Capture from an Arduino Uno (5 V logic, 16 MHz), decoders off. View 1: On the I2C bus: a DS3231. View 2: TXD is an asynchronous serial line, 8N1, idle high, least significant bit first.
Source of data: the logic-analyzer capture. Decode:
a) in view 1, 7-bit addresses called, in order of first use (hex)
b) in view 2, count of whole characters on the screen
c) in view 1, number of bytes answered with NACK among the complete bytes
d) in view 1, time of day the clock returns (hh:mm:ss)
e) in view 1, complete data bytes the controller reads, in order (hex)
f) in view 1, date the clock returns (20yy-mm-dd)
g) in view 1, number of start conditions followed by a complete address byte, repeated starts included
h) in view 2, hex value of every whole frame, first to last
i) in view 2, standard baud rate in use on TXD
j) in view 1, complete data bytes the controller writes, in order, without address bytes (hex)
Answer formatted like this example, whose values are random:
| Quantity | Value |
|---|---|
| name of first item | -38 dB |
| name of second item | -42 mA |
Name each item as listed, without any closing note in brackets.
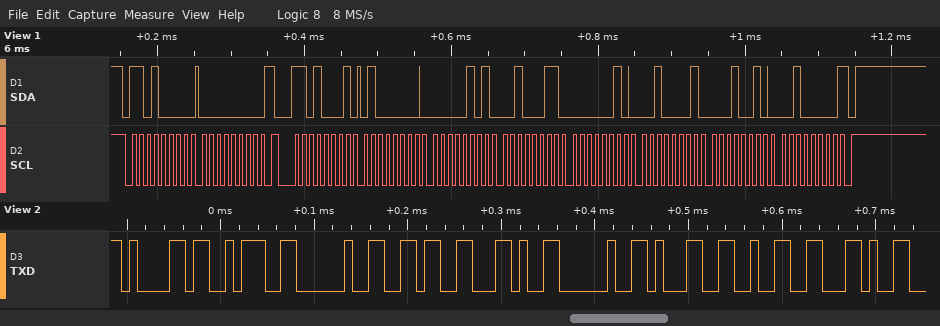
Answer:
| Quantity | Value |
|---|---|
| in view 1, 7-bit addresses called, in order of first use | 0x68 |
| in view 2, count of whole characters on the screen | 9 |
| in view 1, number of bytes answered with NACK among the complete bytes | 1 |
| in view 1, time of day the clock returns | 23:05:40 |
| in view 1, complete data bytes the controller reads, in order | 40 05 23 02 21 12 20 |
| in view 1, date the clock returns | 2020-12-21 |
| in view 1, number of start conditions followed by a complete address byte, repeated starts included | 2 |
| in view 2, hex value of every whole frame, first to last | 61 3A 20 36 2C 20 31 32 2C |
| in view 2, standard baud rate in use on TXD | 115200 baud |
| in view 1, complete data bytes the controller writes, in order, without address bytes | 00 |
